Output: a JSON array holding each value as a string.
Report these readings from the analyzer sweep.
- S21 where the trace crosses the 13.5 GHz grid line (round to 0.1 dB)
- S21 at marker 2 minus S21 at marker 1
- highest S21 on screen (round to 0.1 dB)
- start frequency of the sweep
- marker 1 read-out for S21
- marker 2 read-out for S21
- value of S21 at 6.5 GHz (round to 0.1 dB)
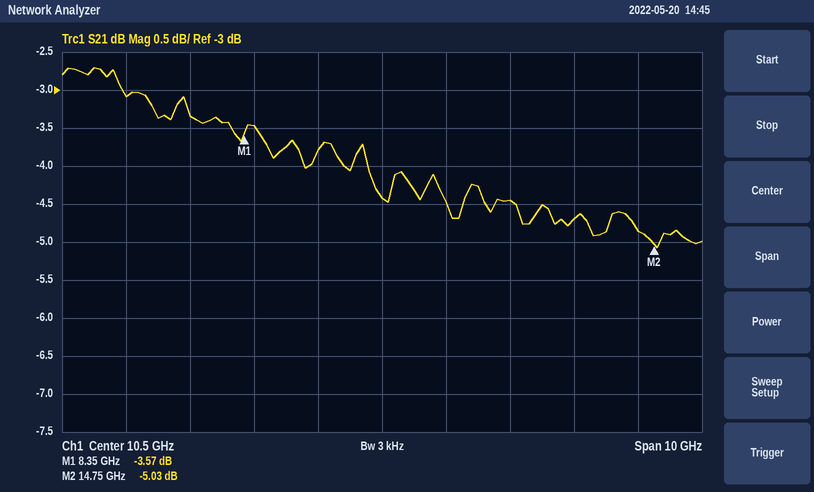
["-4.7 dB", "-1.46 dB", "-2.7 dB", "5.5 GHz", "-3.57 dB", "-5.03 dB", "-3.1 dB"]
